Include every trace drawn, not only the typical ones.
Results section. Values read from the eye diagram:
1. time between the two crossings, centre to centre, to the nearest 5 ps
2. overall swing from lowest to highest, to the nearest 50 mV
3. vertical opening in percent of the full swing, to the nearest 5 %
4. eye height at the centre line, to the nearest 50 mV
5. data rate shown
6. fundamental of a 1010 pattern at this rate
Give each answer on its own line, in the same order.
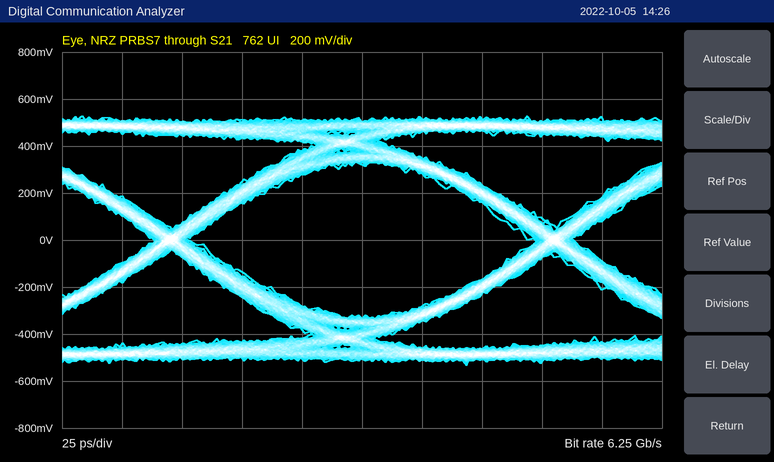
160 ps
1.05 V
60 %
650 mV
6.25 Gb/s
3.125 GHz
